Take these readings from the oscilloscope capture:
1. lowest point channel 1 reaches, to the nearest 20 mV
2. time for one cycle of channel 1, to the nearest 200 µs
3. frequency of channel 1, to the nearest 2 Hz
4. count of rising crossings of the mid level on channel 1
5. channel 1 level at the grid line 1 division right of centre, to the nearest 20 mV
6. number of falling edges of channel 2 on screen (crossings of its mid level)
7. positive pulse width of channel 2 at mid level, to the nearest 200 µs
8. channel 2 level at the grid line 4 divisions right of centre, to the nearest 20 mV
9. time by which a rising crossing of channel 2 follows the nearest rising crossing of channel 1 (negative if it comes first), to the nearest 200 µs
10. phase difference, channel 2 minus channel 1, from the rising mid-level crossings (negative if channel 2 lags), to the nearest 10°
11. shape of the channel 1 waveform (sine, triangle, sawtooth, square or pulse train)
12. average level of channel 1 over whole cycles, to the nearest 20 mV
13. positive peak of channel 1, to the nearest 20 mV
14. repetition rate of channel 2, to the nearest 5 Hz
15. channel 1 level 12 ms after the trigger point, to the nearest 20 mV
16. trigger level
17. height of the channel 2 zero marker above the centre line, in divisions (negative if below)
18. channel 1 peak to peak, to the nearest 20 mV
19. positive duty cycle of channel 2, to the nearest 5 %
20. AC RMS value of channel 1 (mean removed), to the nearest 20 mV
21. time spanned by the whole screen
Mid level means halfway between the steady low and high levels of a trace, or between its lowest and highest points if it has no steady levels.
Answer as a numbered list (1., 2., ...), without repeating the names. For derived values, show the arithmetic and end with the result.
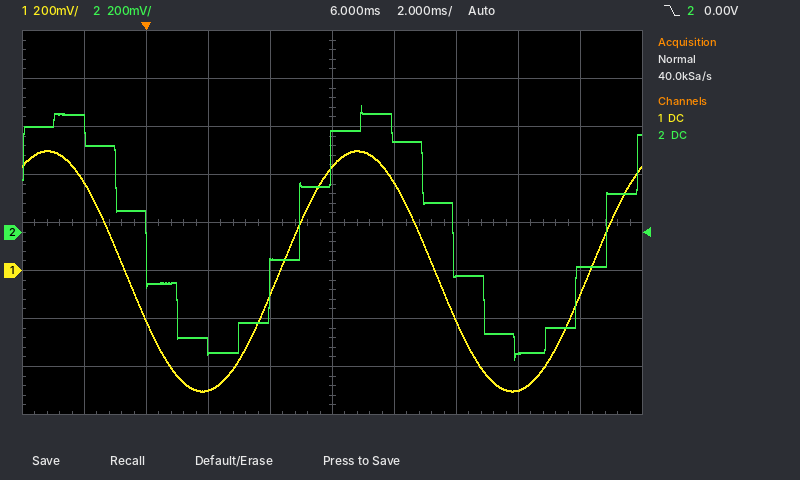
1. -500 mV
2. 10.0 ms
3. 1 / 10.0 ms ≈ 100 Hz
4. 2
5. 360 mV
6. 2
7. 5.0 ms
8. -140 mV
9. +600 µs
10. −360° × (+600 µs) / 10.0 ms ≈ -21.6°, so -20° to the nearest 10°
11. sine
12. (500 mV + (-500 mV)) / 2 ≈ 0 mV
13. 500 mV
14. 100 Hz
15. -500 mV
16. 0.00 V
17. -0.2 div
18. 500 mV − (-500 mV) = 1.00 V
19. 50 %
20. 1.00 V / (2√2) ≈ 354 mV, so 360 mV to the nearest 20 mV
21. 20 ms
